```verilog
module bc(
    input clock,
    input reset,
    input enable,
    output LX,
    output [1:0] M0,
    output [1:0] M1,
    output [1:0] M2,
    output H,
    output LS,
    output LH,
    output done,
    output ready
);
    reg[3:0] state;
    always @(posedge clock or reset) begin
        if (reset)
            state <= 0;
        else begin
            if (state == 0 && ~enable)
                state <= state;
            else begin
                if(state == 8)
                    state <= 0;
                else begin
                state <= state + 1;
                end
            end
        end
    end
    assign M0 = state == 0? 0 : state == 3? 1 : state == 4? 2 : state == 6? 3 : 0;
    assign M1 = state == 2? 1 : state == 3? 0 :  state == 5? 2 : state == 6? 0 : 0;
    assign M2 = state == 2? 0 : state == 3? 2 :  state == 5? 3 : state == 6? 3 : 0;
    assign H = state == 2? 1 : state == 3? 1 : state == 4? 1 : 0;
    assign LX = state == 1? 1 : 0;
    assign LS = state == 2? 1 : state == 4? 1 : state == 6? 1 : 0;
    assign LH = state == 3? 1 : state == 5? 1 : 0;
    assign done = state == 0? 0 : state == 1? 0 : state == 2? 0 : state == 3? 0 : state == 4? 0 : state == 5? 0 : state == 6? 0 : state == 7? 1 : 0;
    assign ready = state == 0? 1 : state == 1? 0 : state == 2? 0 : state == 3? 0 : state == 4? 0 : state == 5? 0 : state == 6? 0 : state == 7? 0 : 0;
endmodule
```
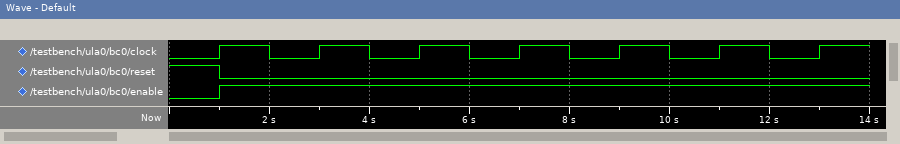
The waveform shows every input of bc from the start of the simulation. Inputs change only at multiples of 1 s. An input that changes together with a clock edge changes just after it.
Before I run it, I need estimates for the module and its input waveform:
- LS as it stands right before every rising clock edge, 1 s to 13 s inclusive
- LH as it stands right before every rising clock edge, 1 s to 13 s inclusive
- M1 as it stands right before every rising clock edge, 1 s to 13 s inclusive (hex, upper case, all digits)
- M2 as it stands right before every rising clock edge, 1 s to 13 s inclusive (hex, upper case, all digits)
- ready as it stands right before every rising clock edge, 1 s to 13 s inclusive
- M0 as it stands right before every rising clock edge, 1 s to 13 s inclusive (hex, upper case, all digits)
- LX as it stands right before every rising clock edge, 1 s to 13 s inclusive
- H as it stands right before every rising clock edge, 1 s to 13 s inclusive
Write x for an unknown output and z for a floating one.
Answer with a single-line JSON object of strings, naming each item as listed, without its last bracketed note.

{"LS as it stands right before every rising clock edge, 1 s to 13 s inclusive": "0 0 1 0 1 0 1", "LH as it stands right before every rising clock edge, 1 s to 13 s inclusive": "0 0 0 1 0 1 0", "M1 as it stands right before every rising clock edge, 1 s to 13 s inclusive": "0, 0, 1, 0, 0, 2, 0", "M2 as it stands right before every rising clock edge, 1 s to 13 s inclusive": "0, 0, 0, 2, 0, 3, 3", "ready as it stands right before every rising clock edge, 1 s to 13 s inclusive": "1 0 0 0 0 0 0", "M0 as it stands right before every rising clock edge, 1 s to 13 s inclusive": "0, 0, 0, 1, 2, 0, 3", "LX as it stands right before every rising clock edge, 1 s to 13 s inclusive": "0 1 0 0 0 0 0", "H as it stands right before every rising clock edge, 1 s to 13 s inclusive": "0 0 1 1 1 0 0"}
